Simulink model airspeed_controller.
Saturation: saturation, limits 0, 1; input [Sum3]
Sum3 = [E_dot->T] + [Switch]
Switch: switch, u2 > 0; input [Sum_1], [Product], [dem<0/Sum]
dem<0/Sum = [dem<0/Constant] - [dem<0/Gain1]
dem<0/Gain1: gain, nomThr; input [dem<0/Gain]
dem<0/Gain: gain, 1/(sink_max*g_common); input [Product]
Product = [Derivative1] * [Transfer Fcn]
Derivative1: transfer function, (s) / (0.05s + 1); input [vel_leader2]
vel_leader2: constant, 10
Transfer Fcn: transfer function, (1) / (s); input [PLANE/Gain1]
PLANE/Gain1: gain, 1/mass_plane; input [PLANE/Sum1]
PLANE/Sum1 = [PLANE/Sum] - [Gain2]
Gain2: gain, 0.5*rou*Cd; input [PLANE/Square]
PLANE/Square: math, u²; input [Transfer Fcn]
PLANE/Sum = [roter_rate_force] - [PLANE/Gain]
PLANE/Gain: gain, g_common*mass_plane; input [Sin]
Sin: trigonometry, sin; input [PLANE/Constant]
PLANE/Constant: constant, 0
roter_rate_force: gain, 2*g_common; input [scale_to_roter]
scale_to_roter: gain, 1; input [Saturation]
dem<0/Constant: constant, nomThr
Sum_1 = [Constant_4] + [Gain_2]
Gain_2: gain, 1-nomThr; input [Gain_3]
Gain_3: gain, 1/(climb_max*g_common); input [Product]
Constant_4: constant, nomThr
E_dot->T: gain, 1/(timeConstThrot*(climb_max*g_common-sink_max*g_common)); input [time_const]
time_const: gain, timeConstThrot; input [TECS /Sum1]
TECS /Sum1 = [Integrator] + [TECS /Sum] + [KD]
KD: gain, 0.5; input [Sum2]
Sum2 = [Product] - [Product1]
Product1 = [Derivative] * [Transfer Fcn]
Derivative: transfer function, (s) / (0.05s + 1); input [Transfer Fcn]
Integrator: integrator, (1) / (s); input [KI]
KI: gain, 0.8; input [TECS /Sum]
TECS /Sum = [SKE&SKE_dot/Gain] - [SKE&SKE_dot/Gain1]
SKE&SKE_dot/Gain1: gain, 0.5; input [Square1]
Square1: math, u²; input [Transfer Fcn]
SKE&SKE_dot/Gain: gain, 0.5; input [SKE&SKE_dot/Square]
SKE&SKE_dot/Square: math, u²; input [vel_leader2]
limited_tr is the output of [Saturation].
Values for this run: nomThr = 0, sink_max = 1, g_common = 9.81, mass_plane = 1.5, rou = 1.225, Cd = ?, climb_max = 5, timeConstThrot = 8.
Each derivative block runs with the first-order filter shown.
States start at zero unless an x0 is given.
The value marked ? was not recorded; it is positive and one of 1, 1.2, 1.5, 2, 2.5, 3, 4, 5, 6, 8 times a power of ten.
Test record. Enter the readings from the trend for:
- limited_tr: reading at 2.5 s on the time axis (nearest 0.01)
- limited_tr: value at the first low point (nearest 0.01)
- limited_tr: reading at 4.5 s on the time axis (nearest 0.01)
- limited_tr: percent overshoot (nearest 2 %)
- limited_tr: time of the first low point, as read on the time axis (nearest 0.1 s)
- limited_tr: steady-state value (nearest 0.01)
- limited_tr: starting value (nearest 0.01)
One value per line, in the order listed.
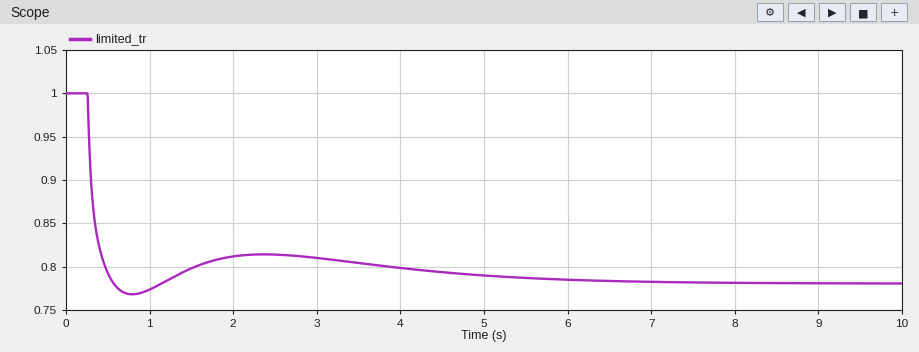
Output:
0.81
0.77
0.79
6 %
0.8 s
0.78
1.00
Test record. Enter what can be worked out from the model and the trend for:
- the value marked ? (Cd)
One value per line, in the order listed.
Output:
0.25
